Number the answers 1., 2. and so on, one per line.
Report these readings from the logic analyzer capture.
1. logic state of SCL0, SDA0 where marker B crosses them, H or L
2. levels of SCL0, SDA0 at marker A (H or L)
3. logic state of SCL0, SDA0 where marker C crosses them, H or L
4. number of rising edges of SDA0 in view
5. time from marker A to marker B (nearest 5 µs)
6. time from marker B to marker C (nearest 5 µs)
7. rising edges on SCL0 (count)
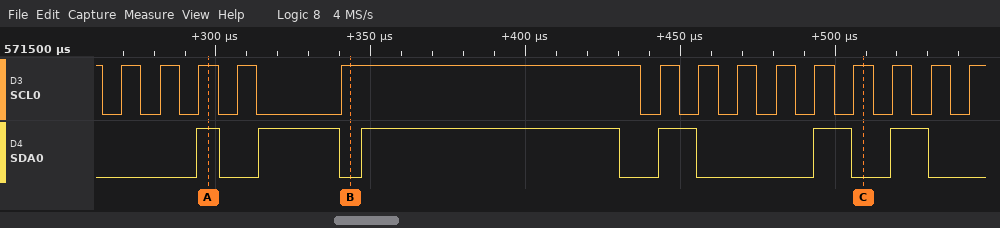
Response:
1. SCL0=H, SDA0=L
2. SCL0=H, SDA0=H
3. SCL0=H, SDA0=L
4. 6
5. 45 µs
6. 165 µs
7. 14
